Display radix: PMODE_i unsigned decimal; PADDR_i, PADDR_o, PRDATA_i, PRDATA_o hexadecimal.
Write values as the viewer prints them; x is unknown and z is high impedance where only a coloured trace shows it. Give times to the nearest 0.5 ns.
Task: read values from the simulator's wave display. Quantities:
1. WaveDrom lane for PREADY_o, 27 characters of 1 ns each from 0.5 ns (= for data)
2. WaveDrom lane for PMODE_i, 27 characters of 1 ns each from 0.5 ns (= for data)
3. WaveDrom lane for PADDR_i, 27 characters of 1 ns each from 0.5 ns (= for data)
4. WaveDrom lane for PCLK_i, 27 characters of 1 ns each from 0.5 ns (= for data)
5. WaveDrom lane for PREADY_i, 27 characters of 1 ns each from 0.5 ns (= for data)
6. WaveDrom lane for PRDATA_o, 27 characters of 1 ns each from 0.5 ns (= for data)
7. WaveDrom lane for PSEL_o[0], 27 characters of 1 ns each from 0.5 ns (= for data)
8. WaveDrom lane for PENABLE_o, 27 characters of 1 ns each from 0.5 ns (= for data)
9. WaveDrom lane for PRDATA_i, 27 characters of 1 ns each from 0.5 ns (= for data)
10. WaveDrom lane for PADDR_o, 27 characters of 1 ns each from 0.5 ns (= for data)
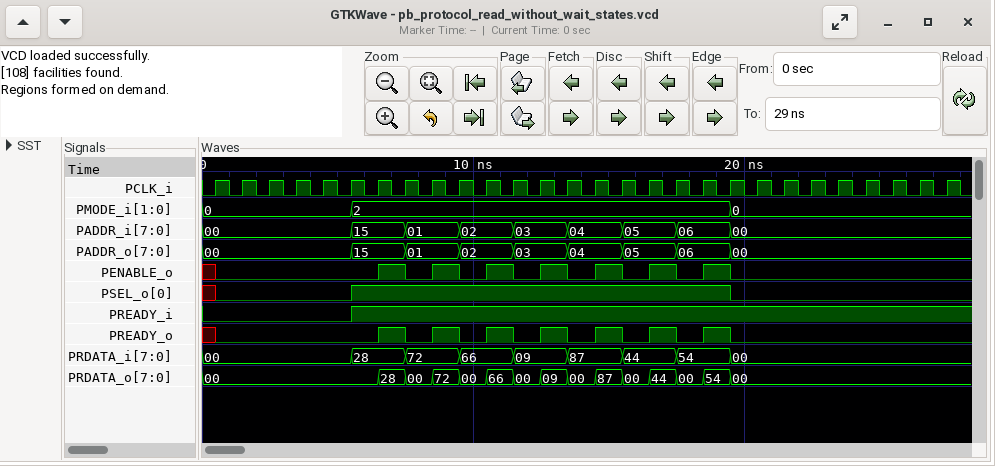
{name: 'PREADY_o', wave: '0.....10101010101010.......'}
{name: 'PMODE_i', wave: '=....=.............=.......', data: '0 2 0'}
{name: 'PADDR_i', wave: '=....=.=.=.=.=.=.=.=.......', data: '00 15 01 02 03 04 05 06 00'}
{name: 'PCLK_i', wave: 'p..........................'}
{name: 'PREADY_i', wave: '0....1.....................'}
{name: 'PRDATA_o', wave: '=.....==============.......', data: '00 28 00 72 00 66 00 09 00 87 00 44 00 54 00'}
{name: 'PSEL_o[0]', wave: '0....1.............0.......'}
{name: 'PENABLE_o', wave: '0.....10101010101010.......'}
{name: 'PRDATA_i', wave: '=....=.=.=.=.=.=.=.=.......', data: '00 28 72 66 09 87 44 54 00'}
{name: 'PADDR_o', wave: '=....=.=.=.=.=.=.=.=.......', data: '00 15 01 02 03 04 05 06 00'}
